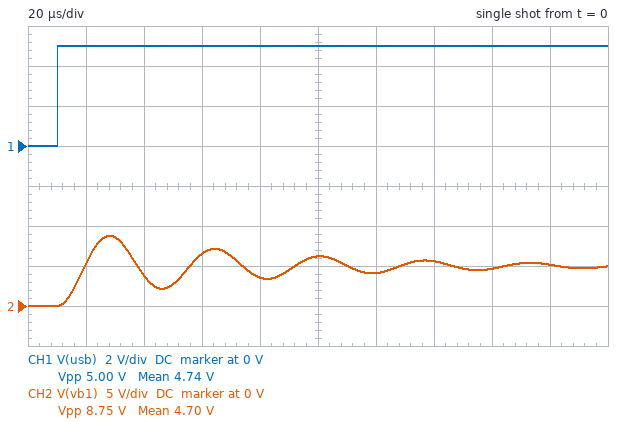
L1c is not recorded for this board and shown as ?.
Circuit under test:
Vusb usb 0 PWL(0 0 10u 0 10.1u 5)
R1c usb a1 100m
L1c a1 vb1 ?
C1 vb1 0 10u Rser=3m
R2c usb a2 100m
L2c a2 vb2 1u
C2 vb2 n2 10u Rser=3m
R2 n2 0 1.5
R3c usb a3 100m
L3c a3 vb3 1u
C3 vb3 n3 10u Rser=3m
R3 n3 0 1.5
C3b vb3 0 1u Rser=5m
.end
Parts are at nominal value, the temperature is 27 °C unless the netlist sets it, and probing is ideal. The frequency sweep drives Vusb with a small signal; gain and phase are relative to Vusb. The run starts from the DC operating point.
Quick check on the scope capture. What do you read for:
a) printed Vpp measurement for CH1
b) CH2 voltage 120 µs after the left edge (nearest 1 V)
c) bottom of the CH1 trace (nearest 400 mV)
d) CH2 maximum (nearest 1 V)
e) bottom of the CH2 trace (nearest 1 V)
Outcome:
5.00 V
4 V
0 V
9 V
0 V
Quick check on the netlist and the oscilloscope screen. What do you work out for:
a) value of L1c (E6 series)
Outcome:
3.3 µH
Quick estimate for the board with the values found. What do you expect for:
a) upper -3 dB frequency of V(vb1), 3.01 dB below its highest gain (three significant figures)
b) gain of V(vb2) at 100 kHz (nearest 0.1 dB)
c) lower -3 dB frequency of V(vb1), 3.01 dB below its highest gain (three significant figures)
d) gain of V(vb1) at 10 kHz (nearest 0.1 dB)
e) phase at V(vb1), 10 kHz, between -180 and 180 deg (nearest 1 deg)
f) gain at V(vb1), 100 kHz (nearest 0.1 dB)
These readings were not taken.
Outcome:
29.9 kHz
-0.9 dB
24.9 kHz
1.2 dB
-4 deg
-21.6 dB
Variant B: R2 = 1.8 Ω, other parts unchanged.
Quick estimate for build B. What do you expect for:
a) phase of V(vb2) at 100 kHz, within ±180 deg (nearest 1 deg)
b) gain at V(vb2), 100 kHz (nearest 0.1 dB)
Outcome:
-19 deg
-0.7 dB
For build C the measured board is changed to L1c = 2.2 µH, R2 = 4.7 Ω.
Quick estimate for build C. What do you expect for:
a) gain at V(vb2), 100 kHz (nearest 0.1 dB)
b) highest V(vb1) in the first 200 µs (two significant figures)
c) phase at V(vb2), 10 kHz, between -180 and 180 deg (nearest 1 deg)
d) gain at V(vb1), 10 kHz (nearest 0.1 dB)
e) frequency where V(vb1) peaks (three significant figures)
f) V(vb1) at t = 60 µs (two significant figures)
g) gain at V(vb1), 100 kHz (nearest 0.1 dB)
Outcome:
-0.2 dB
8.5 V
-1 deg
0.8 dB
33.5 kHz
5.8 V
-17.7 dB
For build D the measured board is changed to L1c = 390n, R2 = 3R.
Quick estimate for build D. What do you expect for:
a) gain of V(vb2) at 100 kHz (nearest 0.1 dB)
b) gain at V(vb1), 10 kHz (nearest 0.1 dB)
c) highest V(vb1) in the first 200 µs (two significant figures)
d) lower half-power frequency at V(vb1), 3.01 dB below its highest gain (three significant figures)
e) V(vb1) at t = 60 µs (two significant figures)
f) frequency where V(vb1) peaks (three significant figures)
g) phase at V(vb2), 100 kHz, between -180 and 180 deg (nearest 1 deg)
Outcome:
-0.4 dB
0.1 dB
7.1 V
48.4 kHz
5.0 V
74.9 kHz
-12 deg
